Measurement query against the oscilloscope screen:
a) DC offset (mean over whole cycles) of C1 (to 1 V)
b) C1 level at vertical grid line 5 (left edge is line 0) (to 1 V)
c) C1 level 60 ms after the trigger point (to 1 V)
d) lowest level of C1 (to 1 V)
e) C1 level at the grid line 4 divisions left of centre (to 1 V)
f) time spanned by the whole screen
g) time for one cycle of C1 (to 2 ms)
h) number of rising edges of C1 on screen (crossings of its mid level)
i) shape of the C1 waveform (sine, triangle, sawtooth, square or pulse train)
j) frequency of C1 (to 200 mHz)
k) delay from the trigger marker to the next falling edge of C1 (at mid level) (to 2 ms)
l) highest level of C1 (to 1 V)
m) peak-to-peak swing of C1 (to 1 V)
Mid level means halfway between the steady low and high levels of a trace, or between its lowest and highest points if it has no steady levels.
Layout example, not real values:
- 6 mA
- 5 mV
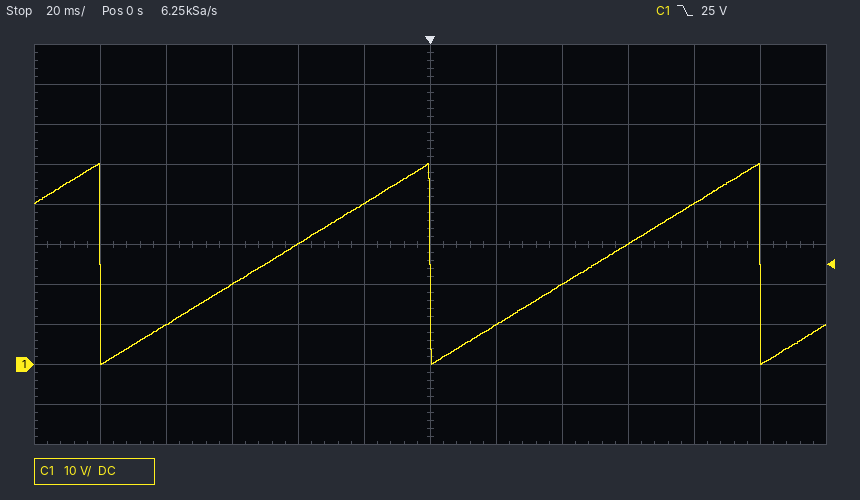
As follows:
- 25 V
- 40 V
- 30 V
- 0 V
- 10 V
- 240 ms
- 100 ms
- 2
- sawtooth
- 10.0 Hz
- 100 ms
- 50 V
- 50 V
